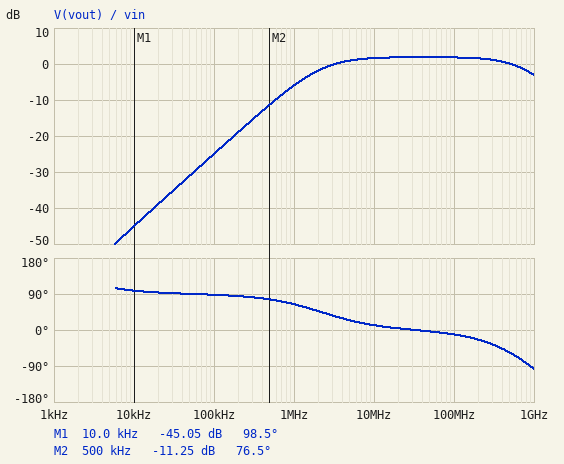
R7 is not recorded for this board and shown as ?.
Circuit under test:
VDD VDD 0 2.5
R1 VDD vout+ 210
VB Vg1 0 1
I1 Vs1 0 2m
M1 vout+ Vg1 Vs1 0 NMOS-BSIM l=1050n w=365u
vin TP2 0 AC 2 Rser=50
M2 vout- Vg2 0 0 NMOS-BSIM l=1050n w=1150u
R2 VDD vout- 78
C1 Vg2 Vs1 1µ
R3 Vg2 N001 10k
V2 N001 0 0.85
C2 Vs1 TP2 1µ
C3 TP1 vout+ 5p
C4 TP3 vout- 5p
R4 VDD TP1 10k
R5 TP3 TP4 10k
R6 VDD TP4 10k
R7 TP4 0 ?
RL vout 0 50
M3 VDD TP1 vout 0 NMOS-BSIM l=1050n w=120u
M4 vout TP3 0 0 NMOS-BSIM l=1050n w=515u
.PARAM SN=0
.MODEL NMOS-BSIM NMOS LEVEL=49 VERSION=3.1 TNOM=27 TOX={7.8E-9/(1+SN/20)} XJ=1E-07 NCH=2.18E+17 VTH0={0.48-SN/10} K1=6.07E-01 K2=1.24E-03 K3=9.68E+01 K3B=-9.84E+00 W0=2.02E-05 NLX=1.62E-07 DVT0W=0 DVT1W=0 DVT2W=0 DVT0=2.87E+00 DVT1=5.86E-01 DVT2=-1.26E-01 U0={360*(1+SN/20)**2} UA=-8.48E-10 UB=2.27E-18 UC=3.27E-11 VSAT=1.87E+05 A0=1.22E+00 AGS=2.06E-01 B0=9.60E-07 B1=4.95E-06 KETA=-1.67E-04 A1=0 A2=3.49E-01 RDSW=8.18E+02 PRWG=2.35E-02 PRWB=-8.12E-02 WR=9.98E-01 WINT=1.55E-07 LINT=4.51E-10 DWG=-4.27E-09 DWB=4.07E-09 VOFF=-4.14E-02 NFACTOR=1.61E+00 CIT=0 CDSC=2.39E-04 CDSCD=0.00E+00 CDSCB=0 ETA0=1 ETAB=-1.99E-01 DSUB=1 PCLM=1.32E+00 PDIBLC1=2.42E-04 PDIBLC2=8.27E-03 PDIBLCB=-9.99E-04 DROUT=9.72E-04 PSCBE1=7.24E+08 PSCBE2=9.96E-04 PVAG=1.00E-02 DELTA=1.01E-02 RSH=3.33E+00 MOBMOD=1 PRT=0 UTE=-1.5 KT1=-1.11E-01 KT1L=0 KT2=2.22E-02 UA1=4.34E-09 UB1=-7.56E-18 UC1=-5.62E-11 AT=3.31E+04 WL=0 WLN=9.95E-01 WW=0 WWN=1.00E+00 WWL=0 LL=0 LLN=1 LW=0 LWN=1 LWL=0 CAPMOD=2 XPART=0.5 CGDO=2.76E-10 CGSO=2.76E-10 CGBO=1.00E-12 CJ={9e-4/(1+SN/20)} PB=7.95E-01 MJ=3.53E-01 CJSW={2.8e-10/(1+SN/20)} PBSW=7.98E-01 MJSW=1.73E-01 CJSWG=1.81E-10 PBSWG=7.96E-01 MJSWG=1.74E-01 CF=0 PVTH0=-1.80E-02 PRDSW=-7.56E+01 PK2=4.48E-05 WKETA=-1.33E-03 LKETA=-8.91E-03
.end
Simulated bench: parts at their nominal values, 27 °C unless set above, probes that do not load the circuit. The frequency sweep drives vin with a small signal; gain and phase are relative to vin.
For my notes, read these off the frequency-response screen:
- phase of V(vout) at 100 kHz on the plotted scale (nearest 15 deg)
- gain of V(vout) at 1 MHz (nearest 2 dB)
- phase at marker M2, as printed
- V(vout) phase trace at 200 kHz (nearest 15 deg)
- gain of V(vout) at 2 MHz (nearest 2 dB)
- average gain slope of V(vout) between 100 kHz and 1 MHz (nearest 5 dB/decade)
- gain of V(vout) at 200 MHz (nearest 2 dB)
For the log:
90 deg
-6 dB
76.5 deg
90 deg
-2 dB
20 dB/decade
2 dB
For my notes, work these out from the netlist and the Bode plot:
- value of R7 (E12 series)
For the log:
4.7 kΩ
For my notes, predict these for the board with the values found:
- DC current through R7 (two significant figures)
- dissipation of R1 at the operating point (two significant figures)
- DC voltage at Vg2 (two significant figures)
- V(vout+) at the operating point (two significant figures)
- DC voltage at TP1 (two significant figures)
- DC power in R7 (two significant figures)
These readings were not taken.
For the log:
170 µA
840 µW
850 mV
2.1 V
2.5 V
140 µW
